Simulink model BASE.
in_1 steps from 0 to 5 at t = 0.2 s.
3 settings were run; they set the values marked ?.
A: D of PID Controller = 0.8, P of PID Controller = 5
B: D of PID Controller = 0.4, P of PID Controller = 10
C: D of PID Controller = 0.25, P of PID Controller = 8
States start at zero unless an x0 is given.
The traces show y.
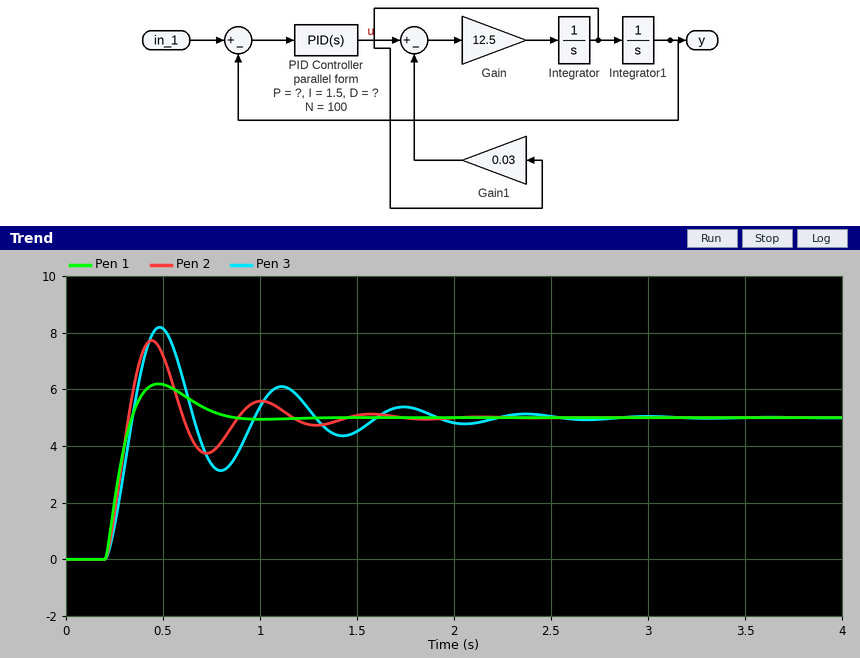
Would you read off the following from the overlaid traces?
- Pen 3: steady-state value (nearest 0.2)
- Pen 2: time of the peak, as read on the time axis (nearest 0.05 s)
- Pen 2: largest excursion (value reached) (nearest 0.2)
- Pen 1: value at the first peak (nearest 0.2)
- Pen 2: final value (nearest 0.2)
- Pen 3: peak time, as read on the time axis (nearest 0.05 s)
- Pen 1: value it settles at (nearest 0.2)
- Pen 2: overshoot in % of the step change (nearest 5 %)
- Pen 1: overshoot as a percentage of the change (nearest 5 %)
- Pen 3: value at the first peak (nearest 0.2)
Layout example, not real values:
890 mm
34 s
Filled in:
5.0
0.45 s
7.8
6.2
5.0
0.50 s
5.0
55 %
25 %
8.2
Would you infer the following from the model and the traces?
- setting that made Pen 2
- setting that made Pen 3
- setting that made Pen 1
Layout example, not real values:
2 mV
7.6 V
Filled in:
B
C
A
